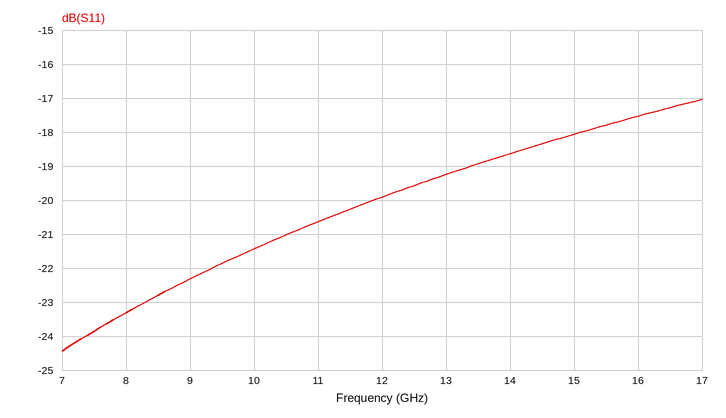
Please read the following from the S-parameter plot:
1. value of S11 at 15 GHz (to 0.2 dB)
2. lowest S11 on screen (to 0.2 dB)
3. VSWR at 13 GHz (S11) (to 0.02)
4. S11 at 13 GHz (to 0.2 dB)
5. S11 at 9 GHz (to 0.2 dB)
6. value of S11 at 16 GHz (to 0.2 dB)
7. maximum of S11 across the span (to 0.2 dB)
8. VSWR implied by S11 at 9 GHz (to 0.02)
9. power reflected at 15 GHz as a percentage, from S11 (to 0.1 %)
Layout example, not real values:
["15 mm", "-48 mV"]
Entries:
["-18.0 dB", "-24.4 dB", "1.24", "-19.2 dB", "-22.4 dB", "-17.6 dB", "-17.0 dB", "1.16", "1.6 %"]
